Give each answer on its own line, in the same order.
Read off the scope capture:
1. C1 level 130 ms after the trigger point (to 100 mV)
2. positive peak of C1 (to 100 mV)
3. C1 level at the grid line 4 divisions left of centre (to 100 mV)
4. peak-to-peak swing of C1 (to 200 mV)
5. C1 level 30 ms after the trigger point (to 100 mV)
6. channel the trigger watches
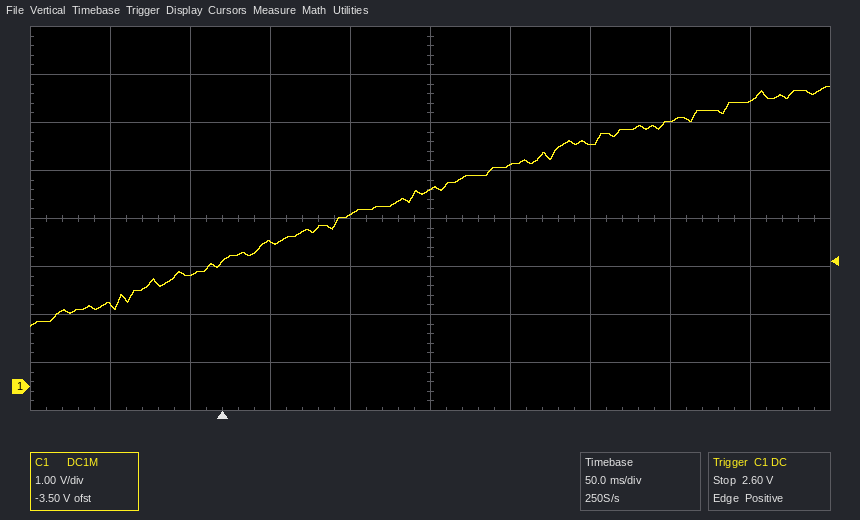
4.1 V
6.2 V
1.7 V
5.0 V
3.0 V
C1
